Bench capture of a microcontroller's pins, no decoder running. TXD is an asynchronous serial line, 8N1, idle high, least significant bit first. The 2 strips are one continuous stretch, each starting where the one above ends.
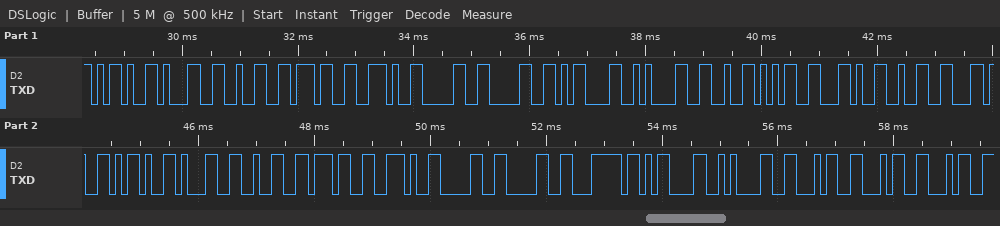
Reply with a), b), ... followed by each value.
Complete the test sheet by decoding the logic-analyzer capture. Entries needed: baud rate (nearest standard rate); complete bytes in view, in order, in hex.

a) 9600 baud
b) 2D 31 32 37 2E 30 30 0D 0A 26 35 2C 32 2C 2D 31 32 37 2E 30 30 7C 0D 0A 46 46 46
